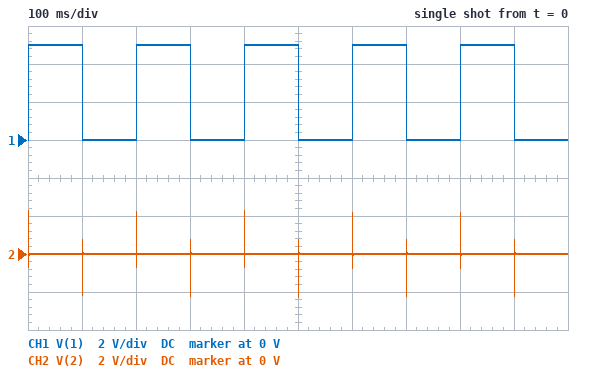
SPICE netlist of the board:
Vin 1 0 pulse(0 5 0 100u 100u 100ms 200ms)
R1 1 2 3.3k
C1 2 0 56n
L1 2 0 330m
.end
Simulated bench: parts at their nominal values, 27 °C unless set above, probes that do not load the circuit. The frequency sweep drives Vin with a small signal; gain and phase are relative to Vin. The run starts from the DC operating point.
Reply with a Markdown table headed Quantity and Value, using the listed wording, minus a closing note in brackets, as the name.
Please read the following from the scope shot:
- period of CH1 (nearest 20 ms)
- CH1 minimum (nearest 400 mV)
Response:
| Quantity | Value |
|---|---|
| period of CH1 | 200 ms |
| CH1 minimum | 0 V |
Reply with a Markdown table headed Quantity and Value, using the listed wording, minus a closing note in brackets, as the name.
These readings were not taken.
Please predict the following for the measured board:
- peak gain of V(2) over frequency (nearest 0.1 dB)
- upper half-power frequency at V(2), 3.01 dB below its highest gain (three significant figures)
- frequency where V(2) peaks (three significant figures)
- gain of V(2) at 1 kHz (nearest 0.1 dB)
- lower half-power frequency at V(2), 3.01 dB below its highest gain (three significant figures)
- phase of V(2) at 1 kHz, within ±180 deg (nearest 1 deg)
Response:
| Quantity | Value |
|---|---|
| peak gain of V(2) over frequency | 0 dB |
| upper half-power frequency at V(2), 3.01 dB below its highest gain | 1.68 kHz |
| frequency where V(2) peaks | 1.17 kHz |
| gain of V(2) at 1 kHz | -0.7 dB |
| lower half-power frequency at V(2), 3.01 dB below its highest gain | 817 Hz |
| phase of V(2) at 1 kHz, within ±180 deg | 23 deg |
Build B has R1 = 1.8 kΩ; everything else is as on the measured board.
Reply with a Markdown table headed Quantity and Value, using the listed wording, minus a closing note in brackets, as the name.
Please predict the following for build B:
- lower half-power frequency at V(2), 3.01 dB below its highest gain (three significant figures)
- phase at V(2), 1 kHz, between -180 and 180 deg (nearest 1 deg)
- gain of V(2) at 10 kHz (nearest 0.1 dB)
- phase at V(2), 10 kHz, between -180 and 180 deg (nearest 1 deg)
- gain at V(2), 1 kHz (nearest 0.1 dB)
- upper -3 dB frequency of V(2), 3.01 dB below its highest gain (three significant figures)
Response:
| Quantity | Value |
|---|---|
| lower half-power frequency at V(2), 3.01 dB below its highest gain | 623 Hz |
| phase at V(2), 1 kHz, between -180 and 180 deg | 13 deg |
| gain of V(2) at 10 kHz | -16.0 dB |
| phase at V(2), 10 kHz, between -180 and 180 deg | -81 deg |
| gain at V(2), 1 kHz | -0.2 dB |
| upper -3 dB frequency of V(2), 3.01 dB below its highest gain | 2.20 kHz |
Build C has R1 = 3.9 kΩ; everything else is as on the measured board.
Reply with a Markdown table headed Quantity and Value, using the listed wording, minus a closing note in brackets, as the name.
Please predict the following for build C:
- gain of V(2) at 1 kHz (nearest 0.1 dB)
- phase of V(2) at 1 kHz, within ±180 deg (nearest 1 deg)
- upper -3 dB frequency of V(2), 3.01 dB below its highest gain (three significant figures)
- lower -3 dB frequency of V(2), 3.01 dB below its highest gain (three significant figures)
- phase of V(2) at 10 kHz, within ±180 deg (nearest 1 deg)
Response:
| Quantity | Value |
|---|---|
| gain of V(2) at 1 kHz | -1.0 dB |
| phase of V(2) at 1 kHz, within ±180 deg | 27 deg |
| upper -3 dB frequency of V(2), 3.01 dB below its highest gain | 1.59 kHz |
| lower -3 dB frequency of V(2), 3.01 dB below its highest gain | 862 Hz |
| phase of V(2) at 10 kHz, within ±180 deg | -86 deg |
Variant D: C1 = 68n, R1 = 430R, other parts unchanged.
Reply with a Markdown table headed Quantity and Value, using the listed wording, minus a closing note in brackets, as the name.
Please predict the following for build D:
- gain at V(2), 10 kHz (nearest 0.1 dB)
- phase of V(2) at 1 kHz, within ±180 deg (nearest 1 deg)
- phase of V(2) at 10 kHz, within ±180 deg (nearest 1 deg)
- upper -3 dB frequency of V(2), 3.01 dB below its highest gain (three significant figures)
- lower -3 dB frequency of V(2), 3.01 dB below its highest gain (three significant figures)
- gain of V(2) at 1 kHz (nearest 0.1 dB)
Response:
| Quantity | Value |
|---|---|
| gain at V(2), 10 kHz | -6.3 dB |
| phase of V(2) at 1 kHz, within ±180 deg | 1 deg |
| phase of V(2) at 10 kHz, within ±180 deg | -61 deg |
| upper -3 dB frequency of V(2), 3.01 dB below its highest gain | 5.64 kHz |
| lower -3 dB frequency of V(2), 3.01 dB below its highest gain | 200 Hz |
| gain of V(2) at 1 kHz | 0 dB |
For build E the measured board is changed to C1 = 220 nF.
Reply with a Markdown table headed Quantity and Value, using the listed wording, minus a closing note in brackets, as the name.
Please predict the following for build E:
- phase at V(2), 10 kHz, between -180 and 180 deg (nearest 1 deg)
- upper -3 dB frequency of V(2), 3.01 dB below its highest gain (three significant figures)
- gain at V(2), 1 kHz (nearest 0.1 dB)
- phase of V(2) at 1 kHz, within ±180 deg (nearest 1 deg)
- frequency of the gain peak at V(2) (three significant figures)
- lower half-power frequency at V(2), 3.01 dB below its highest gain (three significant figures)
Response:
| Quantity | Value |
|---|---|
| phase at V(2), 10 kHz, between -180 and 180 deg | -89 deg |
| upper -3 dB frequency of V(2), 3.01 dB below its highest gain | 710 Hz |
| gain at V(2), 1 kHz | -9.9 dB |
| phase of V(2) at 1 kHz, within ±180 deg | -71 deg |
| frequency of the gain peak at V(2) | 591 Hz |
| lower half-power frequency at V(2), 3.01 dB below its highest gain | 491 Hz |
